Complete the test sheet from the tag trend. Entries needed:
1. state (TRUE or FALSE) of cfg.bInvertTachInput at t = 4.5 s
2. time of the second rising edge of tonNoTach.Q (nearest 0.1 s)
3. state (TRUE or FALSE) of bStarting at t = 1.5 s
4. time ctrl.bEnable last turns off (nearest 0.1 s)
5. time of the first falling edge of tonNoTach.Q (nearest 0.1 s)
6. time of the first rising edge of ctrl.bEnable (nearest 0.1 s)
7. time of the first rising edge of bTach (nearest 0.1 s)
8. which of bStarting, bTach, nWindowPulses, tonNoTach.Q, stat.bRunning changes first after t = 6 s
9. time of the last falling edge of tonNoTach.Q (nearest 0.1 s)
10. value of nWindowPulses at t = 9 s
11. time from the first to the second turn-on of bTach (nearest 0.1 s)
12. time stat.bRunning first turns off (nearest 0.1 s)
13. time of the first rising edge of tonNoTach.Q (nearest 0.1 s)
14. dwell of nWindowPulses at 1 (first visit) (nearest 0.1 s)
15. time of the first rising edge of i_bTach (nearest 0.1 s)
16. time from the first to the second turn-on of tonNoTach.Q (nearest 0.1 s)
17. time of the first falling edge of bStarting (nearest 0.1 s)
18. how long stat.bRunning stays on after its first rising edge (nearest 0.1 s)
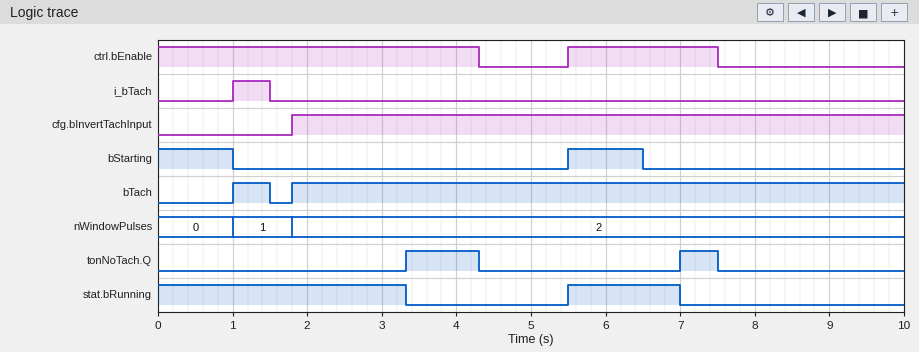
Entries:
TRUE
7.0 s
FALSE
7.5 s
4.3 s
5.5 s
1.0 s
bStarting
7.5 s
2
0.8 s
3.3 s
3.3 s
0.8 s
1.0 s
3.7 s
1.0 s
1.5 s
